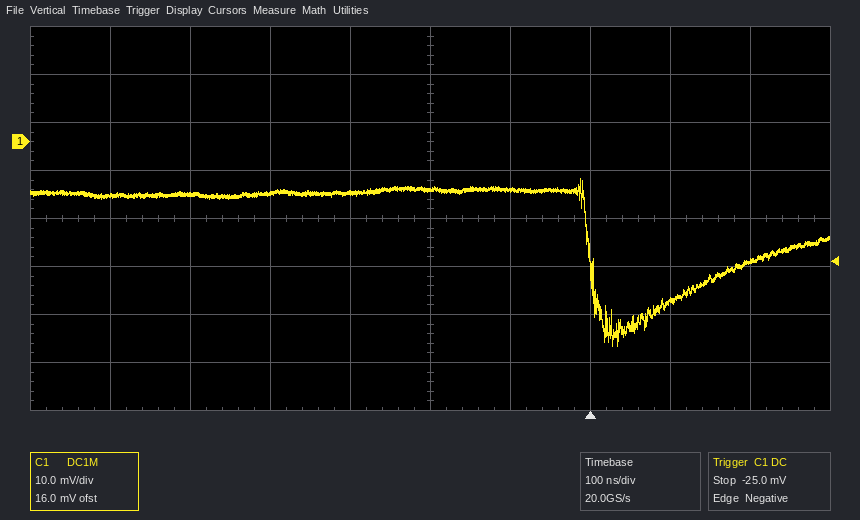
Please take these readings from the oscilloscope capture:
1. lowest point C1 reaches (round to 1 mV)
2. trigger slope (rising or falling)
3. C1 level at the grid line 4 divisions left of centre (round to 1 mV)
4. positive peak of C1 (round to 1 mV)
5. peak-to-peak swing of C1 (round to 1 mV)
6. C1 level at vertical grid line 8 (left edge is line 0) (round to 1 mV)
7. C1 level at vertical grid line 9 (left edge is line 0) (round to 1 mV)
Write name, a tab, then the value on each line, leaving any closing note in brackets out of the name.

lowest point C1 reaches	-43 mV
trigger slope	falling
C1 level at the grid line 4 divisions left of centre	-11 mV
positive peak of C1	-8 mV
peak-to-peak swing of C1	35 mV
C1 level at vertical grid line 8 (left edge is line 0)	-33 mV
C1 level at vertical grid line 9 (left edge is line 0)	-25 mV
